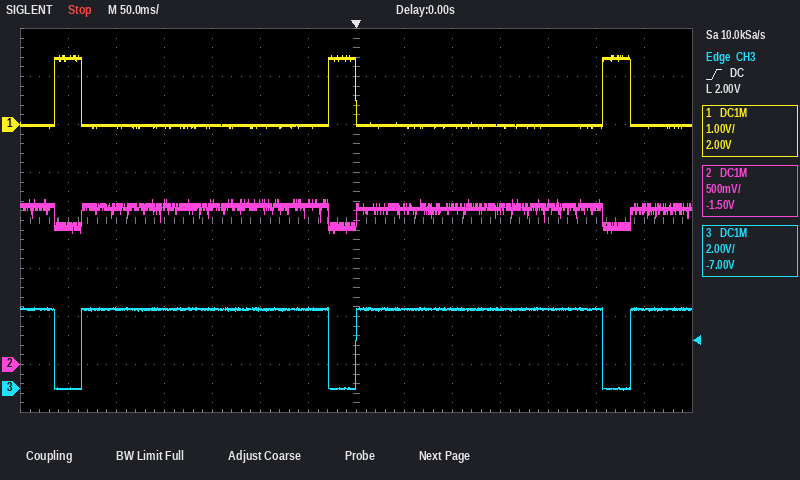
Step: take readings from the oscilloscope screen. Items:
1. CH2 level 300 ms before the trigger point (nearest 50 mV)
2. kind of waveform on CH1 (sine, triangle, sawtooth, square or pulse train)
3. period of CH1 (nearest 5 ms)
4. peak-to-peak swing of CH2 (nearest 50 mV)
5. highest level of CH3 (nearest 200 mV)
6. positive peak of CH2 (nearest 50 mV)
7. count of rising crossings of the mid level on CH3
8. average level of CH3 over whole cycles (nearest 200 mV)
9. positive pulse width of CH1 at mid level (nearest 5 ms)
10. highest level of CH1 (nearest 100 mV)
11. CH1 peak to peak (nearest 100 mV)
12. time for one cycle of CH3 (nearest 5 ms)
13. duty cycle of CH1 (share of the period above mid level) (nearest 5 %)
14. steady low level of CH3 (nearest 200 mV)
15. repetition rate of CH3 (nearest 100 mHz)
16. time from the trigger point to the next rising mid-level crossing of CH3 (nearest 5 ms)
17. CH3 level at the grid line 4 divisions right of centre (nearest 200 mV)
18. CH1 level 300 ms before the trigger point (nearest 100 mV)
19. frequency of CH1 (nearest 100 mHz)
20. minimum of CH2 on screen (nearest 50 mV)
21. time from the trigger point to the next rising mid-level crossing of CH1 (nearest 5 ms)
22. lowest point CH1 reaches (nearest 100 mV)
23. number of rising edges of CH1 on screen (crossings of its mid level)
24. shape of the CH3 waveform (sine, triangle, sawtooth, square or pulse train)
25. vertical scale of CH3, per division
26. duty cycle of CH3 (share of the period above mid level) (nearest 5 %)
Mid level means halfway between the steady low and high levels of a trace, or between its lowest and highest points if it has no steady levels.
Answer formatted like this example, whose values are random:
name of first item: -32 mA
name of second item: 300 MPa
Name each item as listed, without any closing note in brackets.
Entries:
CH2 level 300 ms before the trigger point: 1.45 V
kind of waveform on CH1: pulse train
period of CH1: 285 ms
peak-to-peak swing of CH2: 350 mV
highest level of CH3: 3.4 V
positive peak of CH2: 1.70 V
count of rising crossings of the mid level on CH3: 3
average level of CH3 over whole cycles: 3.0 V
positive pulse width of CH1 at mid level: 30 ms
highest level of CH1: 1.4 V
CH1 peak to peak: 1.5 V
time for one cycle of CH3: 285 ms
duty cycle of CH1 (share of the period above mid level): 10 %
steady low level of CH3: 0.0 V
repetition rate of CH3: 3.5 Hz
time from the trigger point to the next rising mid-level crossing of CH3: 285 ms
CH3 level at the grid line 4 divisions right of centre: 3.2 V
CH1 level 300 ms before the trigger point: 1.4 V
frequency of CH1: 3.5 Hz
minimum of CH2 on screen: 1.35 V
time from the trigger point to the next rising mid-level crossing of CH1: 255 ms
lowest point CH1 reaches: -100 mV
number of rising edges of CH1 on screen: 3
shape of the CH3 waveform: pulse train
vertical scale of CH3, per division: 2 V
duty cycle of CH3 (share of the period above mid level): 90 %
